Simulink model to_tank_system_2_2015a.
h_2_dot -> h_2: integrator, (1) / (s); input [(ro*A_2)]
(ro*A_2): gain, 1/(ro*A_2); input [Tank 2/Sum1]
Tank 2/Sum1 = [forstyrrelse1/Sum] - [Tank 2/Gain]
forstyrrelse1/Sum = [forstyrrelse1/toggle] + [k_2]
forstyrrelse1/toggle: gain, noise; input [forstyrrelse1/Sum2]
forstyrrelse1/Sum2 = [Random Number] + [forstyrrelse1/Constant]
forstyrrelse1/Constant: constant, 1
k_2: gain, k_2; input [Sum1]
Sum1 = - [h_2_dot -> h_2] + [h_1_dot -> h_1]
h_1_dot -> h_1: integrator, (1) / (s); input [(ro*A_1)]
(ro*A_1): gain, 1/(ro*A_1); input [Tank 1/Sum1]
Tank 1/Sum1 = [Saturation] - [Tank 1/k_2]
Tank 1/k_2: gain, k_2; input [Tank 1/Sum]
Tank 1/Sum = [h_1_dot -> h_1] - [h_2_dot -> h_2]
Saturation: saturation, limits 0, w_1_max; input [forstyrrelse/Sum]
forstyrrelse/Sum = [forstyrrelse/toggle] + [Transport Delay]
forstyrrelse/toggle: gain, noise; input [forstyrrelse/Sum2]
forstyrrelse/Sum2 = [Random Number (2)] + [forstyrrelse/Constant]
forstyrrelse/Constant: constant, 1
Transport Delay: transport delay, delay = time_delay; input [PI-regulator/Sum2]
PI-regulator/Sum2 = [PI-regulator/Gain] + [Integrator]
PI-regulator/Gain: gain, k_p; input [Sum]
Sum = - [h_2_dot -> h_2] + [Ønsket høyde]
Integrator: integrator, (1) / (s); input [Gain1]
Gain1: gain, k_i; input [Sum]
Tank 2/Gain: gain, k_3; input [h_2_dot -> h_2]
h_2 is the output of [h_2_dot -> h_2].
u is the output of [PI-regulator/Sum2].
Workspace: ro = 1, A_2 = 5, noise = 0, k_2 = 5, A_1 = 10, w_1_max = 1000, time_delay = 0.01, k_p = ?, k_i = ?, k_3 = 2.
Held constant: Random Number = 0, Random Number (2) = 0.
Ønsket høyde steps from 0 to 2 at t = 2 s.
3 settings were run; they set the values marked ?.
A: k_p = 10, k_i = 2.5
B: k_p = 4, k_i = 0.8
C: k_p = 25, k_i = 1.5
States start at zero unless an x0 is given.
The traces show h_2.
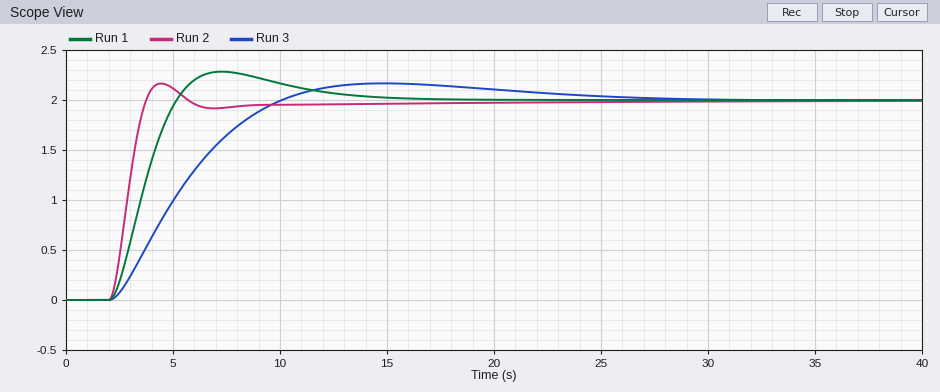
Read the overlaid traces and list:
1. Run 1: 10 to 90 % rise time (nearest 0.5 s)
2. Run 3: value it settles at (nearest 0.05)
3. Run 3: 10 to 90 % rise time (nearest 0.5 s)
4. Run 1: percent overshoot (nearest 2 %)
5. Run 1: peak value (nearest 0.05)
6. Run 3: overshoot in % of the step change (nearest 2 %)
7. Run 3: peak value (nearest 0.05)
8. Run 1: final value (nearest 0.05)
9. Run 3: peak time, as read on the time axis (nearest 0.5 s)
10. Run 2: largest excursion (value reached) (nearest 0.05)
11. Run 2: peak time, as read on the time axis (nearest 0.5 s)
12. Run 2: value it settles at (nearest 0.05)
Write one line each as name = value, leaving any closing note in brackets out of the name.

Run 1: 10 to 90 % rise time = 2.0 s
Run 3: value it settles at = 2.00
Run 3: 10 to 90 % rise time = 5.5 s
Run 1: percent overshoot = 14 %
Run 1: peak value = 2.30
Run 3: overshoot in % of the step change = 8 %
Run 3: peak value = 2.15
Run 1: final value = 2.00
Run 3: peak time, as read on the time axis = 15.0 s
Run 2: largest excursion (value reached) = 2.15
Run 2: peak time, as read on the time axis = 4.5 s
Run 2: value it settles at = 2.00
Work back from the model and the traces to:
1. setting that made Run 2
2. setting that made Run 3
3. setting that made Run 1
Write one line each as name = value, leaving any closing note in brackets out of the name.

setting that made Run 2 = C
setting that made Run 3 = B
setting that made Run 1 = A
